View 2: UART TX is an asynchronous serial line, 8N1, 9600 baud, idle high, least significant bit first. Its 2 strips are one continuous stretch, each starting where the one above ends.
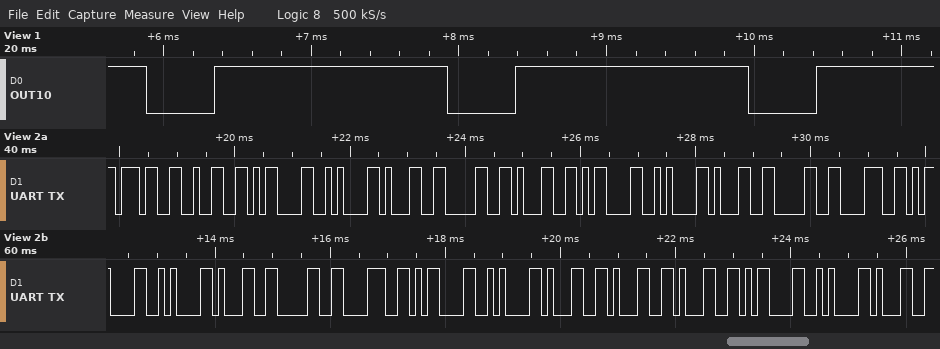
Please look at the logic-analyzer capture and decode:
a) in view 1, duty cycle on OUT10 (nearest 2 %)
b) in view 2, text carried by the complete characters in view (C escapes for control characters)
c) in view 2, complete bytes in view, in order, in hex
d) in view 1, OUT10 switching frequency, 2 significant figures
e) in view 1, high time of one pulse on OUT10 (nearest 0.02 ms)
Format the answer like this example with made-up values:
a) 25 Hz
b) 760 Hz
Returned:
a) 78 %
b) "72\r\n101\r\n108\r\n108\r\n111\r\n1"
c) 0x37 0x32 0x0D 0x0A 0x31 0x30 0x31 0x0D 0x0A 0x31 0x30 0x38 0x0D 0x0A 0x31 0x30 0x38 0x0D 0x0A 0x31 0x31 0x31 0x0D 0x0A 0x31
d) 490 Hz
e) 1.58 ms
